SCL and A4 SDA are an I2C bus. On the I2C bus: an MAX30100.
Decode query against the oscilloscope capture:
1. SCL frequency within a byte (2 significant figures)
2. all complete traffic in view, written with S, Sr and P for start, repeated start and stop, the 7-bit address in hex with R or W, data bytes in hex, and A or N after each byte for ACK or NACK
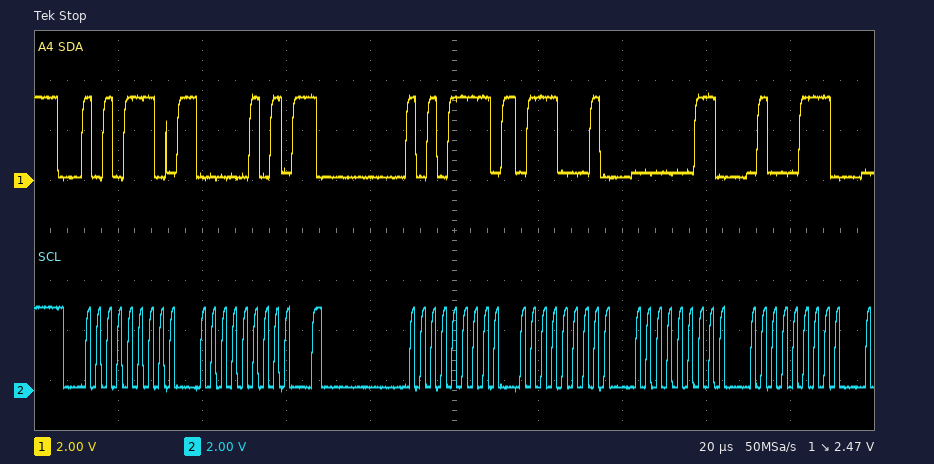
400 kHz
S 57W A 05 A Sr 57R A 71 A 03 A 47 A
